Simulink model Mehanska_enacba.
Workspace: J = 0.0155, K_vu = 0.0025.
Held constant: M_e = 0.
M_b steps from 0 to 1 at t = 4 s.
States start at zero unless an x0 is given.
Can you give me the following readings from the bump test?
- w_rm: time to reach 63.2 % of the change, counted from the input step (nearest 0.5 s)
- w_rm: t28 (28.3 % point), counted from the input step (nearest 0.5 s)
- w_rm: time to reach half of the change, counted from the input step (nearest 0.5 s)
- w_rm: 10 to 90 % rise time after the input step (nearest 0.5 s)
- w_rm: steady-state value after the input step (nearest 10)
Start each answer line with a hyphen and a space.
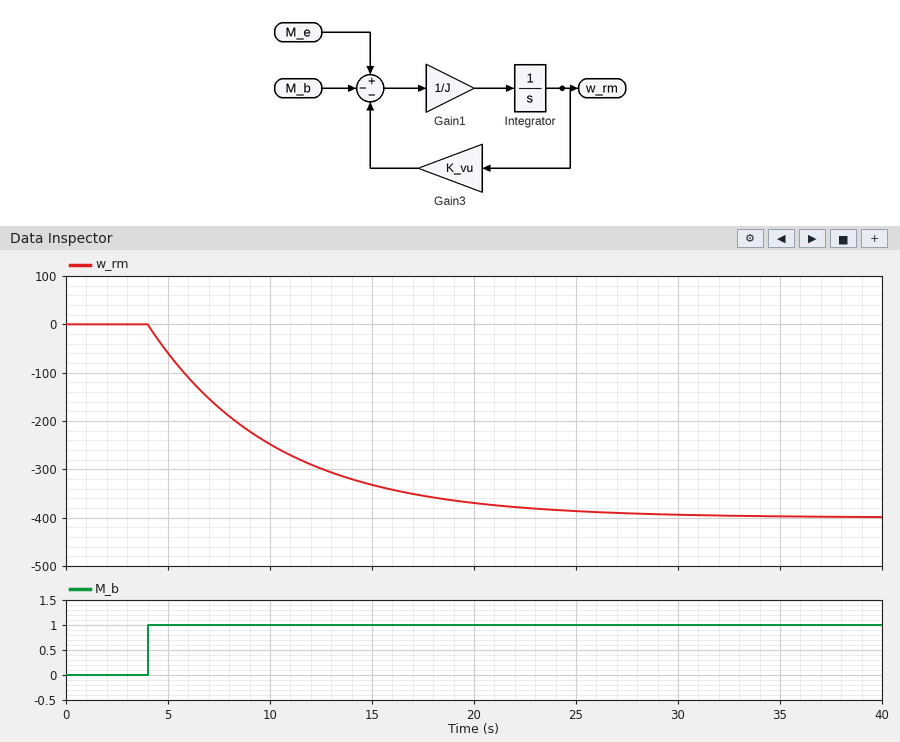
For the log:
- 6.0 s
- 2.0 s
- 4.5 s
- 13.5 s
- -400
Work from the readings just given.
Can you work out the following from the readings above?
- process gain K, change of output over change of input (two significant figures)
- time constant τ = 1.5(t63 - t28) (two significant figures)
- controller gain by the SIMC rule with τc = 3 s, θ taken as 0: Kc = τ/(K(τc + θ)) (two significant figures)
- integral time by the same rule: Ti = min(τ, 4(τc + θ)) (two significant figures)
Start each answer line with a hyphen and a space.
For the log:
- -400
- 6.0 s
- -0.0050
- 6.0 s
